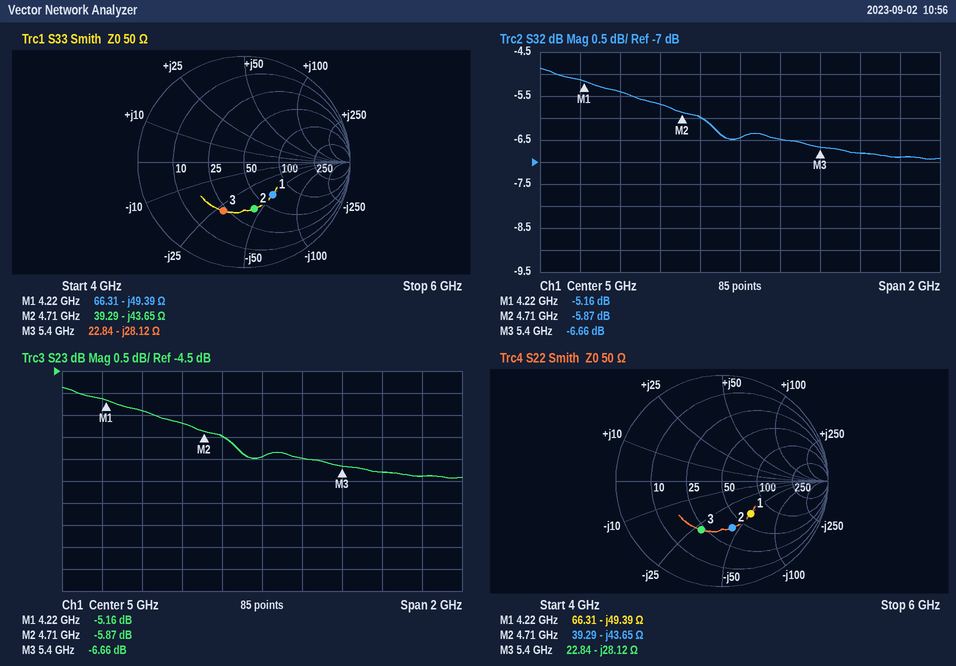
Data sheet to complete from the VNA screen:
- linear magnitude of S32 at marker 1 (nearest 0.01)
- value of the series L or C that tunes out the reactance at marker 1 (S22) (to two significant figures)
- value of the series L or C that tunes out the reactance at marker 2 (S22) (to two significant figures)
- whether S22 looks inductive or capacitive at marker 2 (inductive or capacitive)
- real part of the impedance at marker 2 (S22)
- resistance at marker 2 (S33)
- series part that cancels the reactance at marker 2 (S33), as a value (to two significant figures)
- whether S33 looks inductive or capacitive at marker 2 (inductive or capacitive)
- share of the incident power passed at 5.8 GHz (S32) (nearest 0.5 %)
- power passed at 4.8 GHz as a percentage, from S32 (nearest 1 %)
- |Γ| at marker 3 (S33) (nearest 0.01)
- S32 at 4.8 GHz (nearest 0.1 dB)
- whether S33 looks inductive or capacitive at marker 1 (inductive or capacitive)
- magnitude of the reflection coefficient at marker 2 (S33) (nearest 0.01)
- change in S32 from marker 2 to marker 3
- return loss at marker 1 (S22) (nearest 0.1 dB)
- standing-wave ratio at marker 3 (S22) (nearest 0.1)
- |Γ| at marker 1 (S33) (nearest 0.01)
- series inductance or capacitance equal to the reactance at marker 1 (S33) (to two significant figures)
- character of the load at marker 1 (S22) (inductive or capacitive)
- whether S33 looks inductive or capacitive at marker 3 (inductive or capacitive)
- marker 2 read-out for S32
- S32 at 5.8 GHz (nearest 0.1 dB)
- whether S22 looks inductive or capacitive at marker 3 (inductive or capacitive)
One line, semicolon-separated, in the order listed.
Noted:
0.55; 1.9 nH; 1.5 nH; capacitive; 39.29 Ω; 39.29 Ω; 1.5 nH; capacitive; 20.5 %; 25 %; 0.50; -6.0 dB; capacitive; 0.45; -0.79 dB; 7.7 dB; 3.0; 0.41; 760 fF; capacitive; capacitive; -5.87 dB; -6.9 dB; capacitive
